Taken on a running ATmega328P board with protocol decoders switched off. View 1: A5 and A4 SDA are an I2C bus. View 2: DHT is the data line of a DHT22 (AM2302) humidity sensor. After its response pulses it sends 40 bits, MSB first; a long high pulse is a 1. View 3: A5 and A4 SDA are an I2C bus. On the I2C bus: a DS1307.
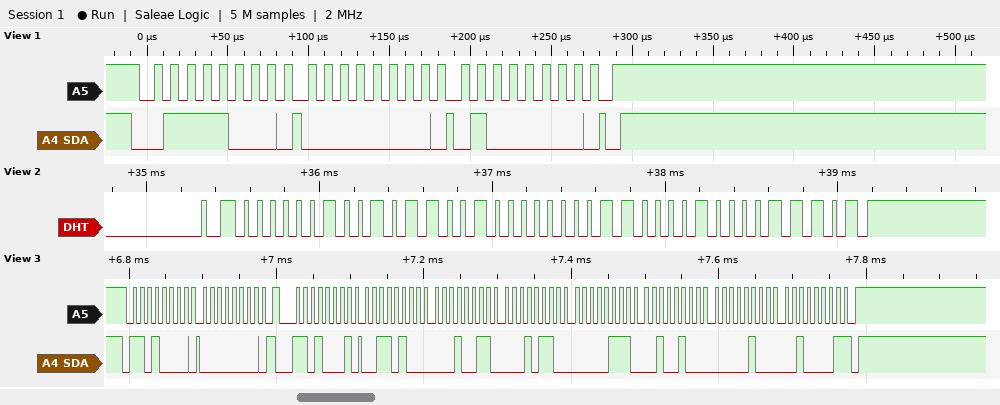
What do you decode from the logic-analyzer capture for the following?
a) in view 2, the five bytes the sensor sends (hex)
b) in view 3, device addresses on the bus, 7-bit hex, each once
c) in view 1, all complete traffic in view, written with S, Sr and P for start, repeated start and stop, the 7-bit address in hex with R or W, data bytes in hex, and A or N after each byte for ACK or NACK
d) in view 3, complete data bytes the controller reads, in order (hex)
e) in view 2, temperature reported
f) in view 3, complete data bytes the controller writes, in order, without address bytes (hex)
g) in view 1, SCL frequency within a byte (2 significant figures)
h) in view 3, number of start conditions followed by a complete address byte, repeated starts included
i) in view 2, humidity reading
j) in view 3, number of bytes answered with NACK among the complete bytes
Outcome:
02 59 00 C2 1D
0x68
S 3CW A 00 A 40 A P
34 13 16 07 24 04 21
19.4 °C
00
100 kHz
2
60.1 %
1
